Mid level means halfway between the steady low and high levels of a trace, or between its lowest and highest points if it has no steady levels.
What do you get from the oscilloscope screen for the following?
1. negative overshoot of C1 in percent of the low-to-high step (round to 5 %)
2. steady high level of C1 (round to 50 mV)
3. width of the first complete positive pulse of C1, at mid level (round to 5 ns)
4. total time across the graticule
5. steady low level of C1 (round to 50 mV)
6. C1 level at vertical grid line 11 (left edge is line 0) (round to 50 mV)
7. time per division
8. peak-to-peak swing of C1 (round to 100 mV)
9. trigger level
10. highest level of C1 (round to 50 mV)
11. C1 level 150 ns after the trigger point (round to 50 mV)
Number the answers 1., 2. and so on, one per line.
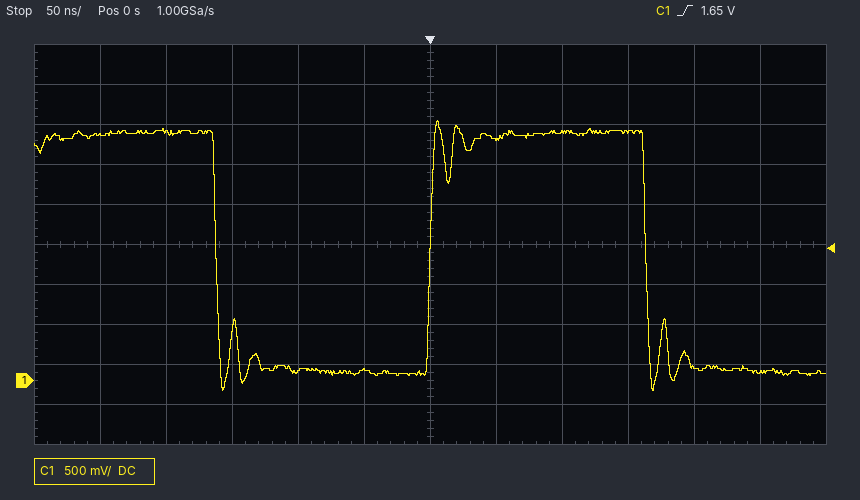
1. 10 %
2. 3.10 V
3. 165 ns
4. 600 ns
5. 100 mV
6. 100 mV
7. 50 ns
8. 3.40 V
9. 1.65 V
10. 3.25 V
11. 3.10 V
